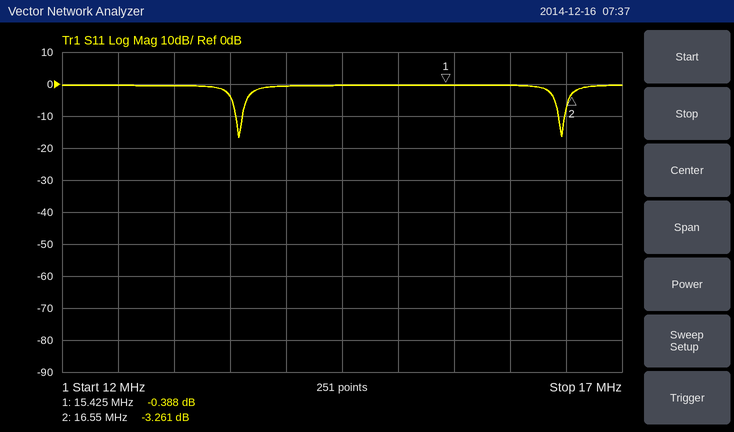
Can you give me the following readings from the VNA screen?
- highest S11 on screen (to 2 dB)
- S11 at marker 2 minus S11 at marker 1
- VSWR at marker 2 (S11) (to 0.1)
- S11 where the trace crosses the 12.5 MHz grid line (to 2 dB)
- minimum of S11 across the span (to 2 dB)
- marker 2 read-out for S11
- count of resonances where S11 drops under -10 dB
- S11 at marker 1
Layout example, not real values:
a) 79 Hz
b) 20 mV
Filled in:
a) 0 dB
b) -2.873 dB
c) 5.4
d) 0 dB
e) -16 dB
f) -3.261 dB
g) 2
h) -0.388 dB
